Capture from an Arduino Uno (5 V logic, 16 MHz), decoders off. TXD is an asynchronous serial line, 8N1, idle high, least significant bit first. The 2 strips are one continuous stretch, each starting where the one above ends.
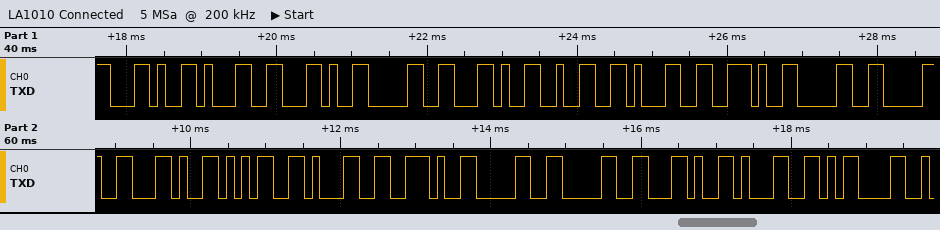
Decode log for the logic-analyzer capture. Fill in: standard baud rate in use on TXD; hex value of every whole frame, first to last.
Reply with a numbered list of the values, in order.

1. 9600 baud
2. 0x2C 0x31 0x2C 0x30 0x2C 0x32 0x31 0x2E 0x30 0x30 0x2C 0x35 0x31 0x2E 0x30 0x30 0x2C 0x31 0x0D
